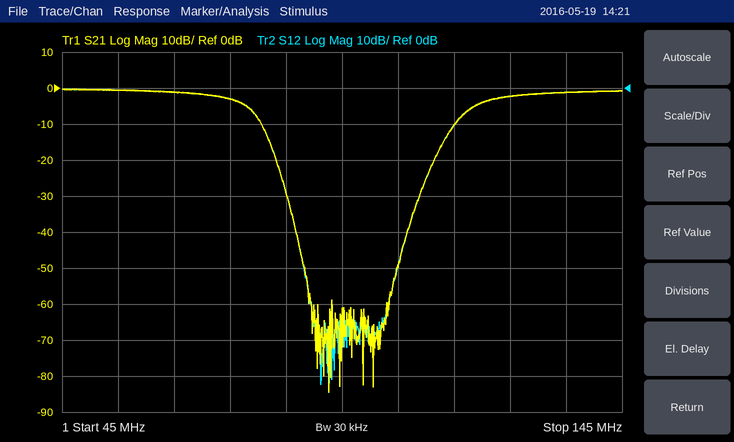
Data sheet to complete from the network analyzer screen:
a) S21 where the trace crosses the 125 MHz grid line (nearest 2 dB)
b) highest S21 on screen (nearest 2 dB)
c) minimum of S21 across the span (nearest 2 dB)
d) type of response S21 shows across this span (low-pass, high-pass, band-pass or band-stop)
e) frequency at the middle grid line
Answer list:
-2 dB
0 dB
-84 dB
band-stop
95 MHz
